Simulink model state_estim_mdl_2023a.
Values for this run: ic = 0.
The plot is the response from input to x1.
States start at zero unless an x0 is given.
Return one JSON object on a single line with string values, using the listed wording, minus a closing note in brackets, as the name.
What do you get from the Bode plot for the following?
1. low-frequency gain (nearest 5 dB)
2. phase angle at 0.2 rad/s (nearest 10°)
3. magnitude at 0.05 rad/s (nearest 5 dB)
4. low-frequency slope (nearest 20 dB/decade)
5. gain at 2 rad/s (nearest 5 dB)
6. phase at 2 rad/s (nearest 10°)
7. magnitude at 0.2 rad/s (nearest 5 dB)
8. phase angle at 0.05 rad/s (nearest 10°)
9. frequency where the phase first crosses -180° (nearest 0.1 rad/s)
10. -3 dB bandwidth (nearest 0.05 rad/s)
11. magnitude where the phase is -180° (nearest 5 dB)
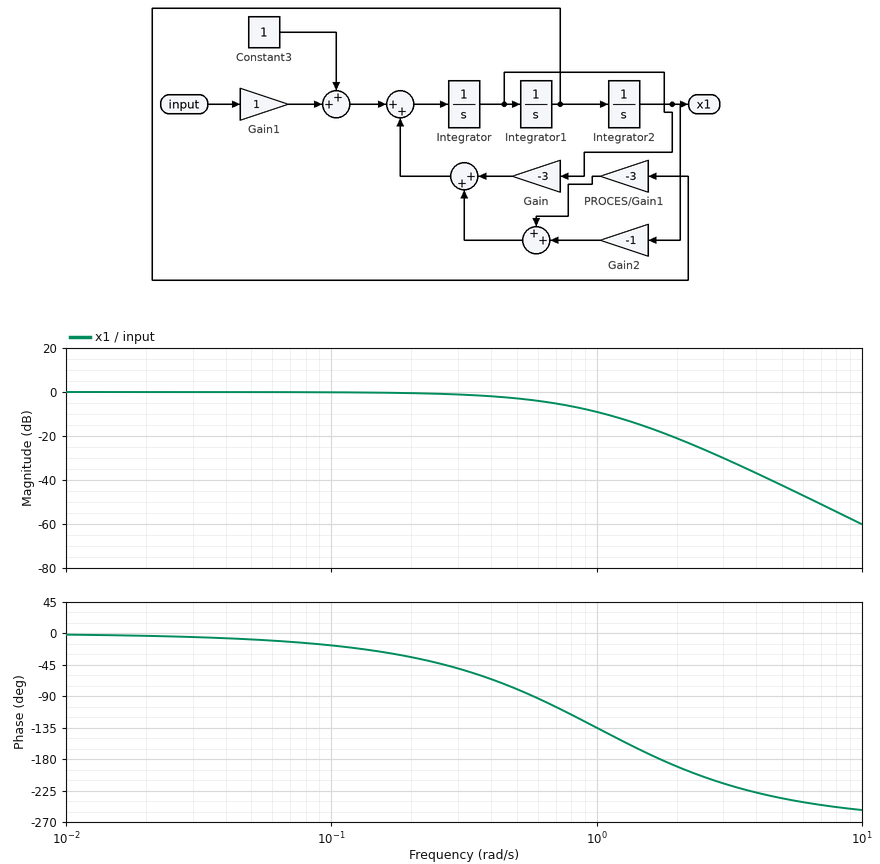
{"low-frequency gain": "0 dB", "phase angle at 0.2 rad/s": "-30°", "magnitude at 0.05 rad/s": "0 dB", "low-frequency slope": "0 dB/decade", "gain at 2 rad/s": "-20 dB", "phase at 2 rad/s": "-190°", "magnitude at 0.2 rad/s": "0 dB", "phase angle at 0.05 rad/s": "-10°", "frequency where the phase first crosses -180°": "1.7 rad/s", "-3 dB bandwidth": "0.50 rad/s", "magnitude where the phase is -180°": "-20 dB"}
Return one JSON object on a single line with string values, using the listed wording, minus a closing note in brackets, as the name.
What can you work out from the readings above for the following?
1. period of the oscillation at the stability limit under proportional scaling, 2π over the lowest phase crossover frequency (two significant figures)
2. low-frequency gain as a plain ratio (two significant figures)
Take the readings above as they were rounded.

{"period of the oscillation at the stability limit under proportional scaling, 2π over the lowest phase crossover frequency": "3.7 s", "low-frequency gain as a plain ratio": "1.0"}
